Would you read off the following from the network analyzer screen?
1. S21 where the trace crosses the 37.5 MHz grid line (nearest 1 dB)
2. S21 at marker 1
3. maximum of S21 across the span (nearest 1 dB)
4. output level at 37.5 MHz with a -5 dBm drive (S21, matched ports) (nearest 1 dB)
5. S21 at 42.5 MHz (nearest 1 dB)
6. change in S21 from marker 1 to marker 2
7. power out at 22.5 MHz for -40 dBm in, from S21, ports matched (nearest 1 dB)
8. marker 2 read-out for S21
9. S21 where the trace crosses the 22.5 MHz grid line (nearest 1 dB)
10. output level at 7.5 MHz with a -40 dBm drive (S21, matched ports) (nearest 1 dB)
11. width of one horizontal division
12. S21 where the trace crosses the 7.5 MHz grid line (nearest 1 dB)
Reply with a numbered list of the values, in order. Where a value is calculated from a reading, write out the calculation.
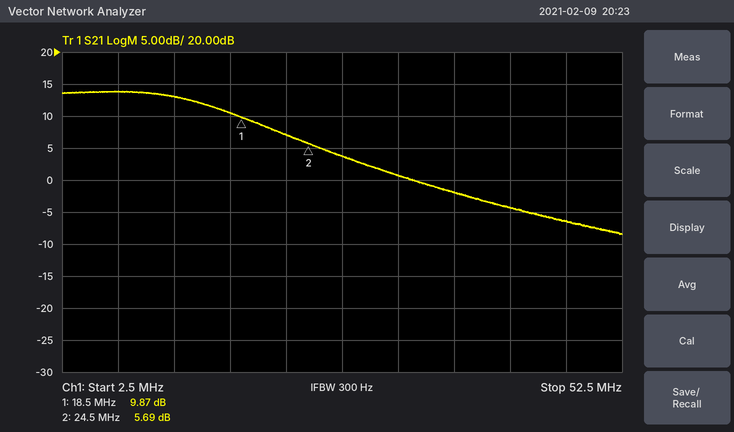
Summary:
1. -2 dB
2. 9.87 dB
3. 14 dB
4. -5 dBm + (-2 dB) = -7 dBm
5. -4 dB
6. 5.69 − (9.87) = -4.18 dB
7. -40 dBm + (7 dB) = -33 dBm
8. 5.69 dB
9. 7 dB
10. -40 dBm + (14 dB) = -26 dBm
11. 5 MHz
12. 14 dB
